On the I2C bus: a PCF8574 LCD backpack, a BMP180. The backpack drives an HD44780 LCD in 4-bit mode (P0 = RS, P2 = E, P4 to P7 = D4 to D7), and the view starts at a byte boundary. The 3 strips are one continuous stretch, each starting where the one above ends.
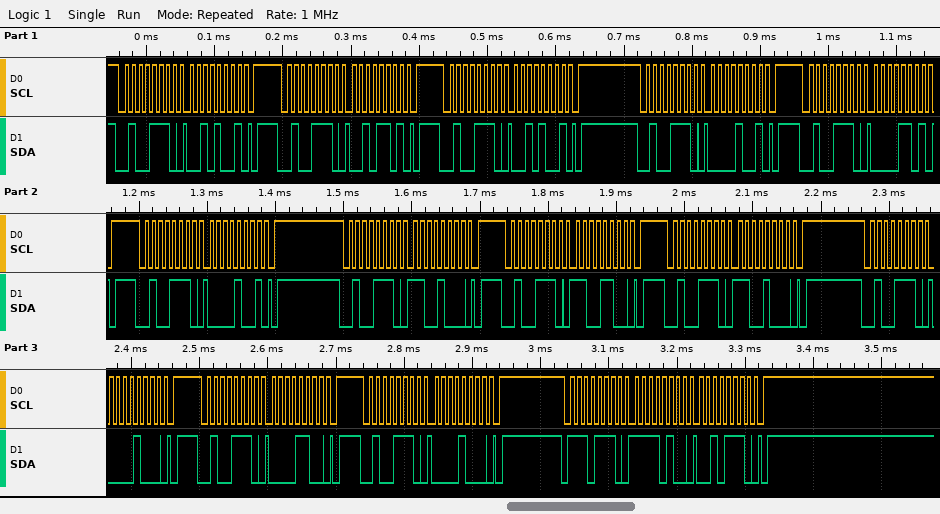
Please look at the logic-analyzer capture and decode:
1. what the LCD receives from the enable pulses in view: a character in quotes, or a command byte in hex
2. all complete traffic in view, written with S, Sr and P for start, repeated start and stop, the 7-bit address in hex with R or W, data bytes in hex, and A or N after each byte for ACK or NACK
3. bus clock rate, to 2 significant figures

' ' 0xC0
S 27W A 29 A P S 27W A 2D A P S 27W A 29 A P S 27W A 09 A P S 27W A 0D A P S 27W A 09 A P S 27W A C8 A P S 27W A CC A P S 27W A C8 A P S 27W A 08 A P S 27W A 0C A P S 27W A 08 A P S 77W A F4 A 2E A P
100 kHz
